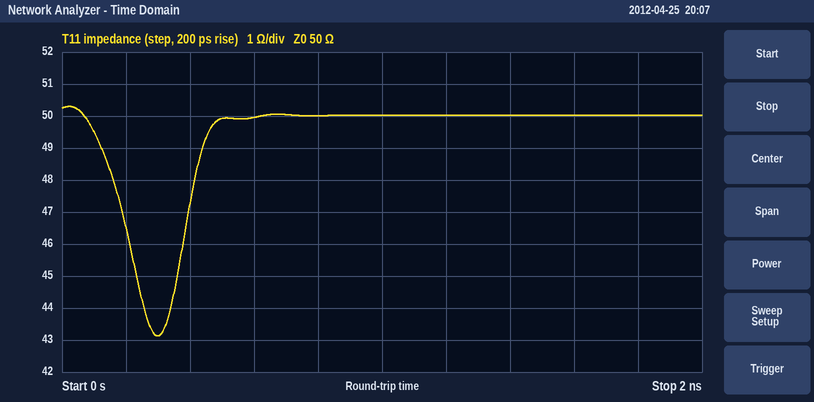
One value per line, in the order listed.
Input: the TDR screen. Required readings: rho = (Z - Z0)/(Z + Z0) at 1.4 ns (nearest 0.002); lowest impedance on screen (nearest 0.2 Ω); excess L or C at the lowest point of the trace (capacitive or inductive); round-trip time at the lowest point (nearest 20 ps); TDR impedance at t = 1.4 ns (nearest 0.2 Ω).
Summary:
0.000
43.2 Ω
capacitive
300 ps
50.0 Ω
